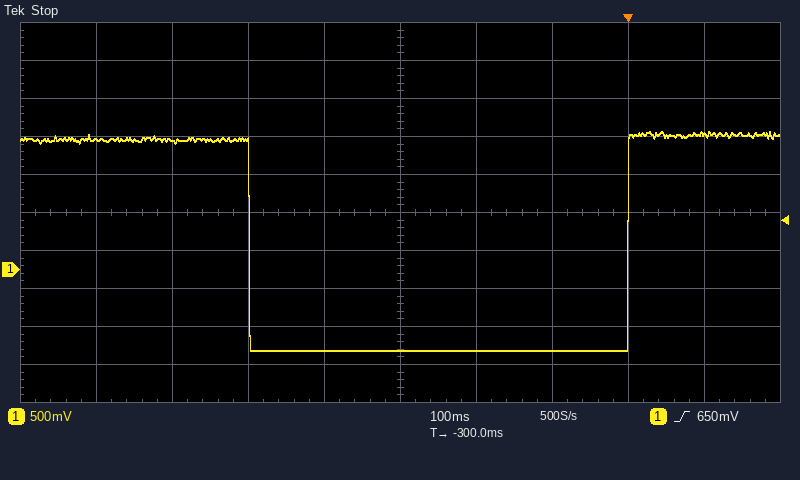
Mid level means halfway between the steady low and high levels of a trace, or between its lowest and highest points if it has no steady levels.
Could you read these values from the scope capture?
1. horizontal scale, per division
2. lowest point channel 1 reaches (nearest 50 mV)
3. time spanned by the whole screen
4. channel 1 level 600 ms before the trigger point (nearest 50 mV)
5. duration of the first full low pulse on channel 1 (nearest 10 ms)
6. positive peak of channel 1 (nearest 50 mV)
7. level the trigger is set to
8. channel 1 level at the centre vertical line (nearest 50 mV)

100 ms
-1.05 V
1 s
1.70 V
500 ms
1.80 V
650 mV
-1.05 V
